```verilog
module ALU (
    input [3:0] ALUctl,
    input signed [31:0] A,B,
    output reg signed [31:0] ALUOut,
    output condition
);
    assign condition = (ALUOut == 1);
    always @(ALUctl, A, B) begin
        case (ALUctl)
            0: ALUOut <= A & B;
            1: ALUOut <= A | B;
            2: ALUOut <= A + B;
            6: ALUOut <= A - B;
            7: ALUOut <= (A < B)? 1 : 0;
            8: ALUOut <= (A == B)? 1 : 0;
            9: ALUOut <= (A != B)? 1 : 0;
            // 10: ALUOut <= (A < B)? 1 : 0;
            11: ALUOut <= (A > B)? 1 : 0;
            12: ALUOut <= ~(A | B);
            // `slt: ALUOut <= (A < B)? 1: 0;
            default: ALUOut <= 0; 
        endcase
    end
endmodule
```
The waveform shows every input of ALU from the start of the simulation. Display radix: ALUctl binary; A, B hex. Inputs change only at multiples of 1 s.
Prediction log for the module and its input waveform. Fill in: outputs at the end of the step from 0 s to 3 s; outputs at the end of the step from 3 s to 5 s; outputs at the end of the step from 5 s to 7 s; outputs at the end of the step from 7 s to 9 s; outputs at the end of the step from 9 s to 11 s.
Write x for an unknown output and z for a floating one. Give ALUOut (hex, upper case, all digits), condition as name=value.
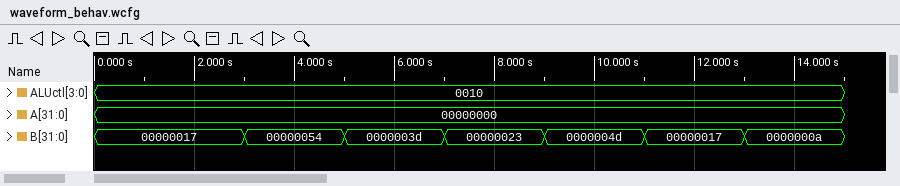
ALUOut=00000017, condition=0
ALUOut=00000054, condition=0
ALUOut=0000003D, condition=0
ALUOut=00000023, condition=0
ALUOut=0000004D, condition=0
